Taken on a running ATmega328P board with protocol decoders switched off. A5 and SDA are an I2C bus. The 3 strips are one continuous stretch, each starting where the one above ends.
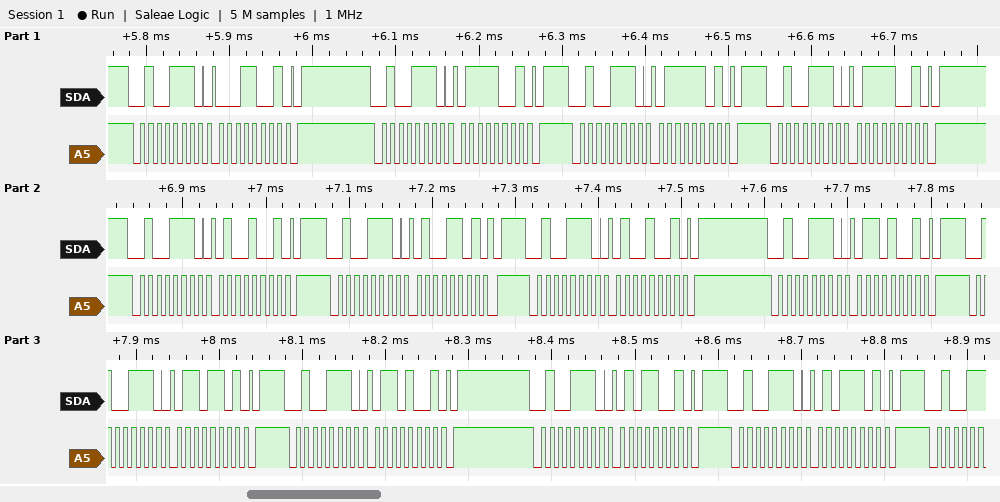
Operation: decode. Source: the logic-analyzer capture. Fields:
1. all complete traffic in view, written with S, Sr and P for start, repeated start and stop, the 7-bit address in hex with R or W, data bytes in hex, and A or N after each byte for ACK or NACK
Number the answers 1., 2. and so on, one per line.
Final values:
1. S 27W A 19 A P S 27W A 79 A P S 27W A 7D A P S 27W A 79 A P S 27W A 49 A P S 27W A 4D A P S 27W A 49 A P S 27W A 69 A P S 27W A 6D A P S 27W A 69 A P S 27W A 59 A P S 27W A 5D A P
